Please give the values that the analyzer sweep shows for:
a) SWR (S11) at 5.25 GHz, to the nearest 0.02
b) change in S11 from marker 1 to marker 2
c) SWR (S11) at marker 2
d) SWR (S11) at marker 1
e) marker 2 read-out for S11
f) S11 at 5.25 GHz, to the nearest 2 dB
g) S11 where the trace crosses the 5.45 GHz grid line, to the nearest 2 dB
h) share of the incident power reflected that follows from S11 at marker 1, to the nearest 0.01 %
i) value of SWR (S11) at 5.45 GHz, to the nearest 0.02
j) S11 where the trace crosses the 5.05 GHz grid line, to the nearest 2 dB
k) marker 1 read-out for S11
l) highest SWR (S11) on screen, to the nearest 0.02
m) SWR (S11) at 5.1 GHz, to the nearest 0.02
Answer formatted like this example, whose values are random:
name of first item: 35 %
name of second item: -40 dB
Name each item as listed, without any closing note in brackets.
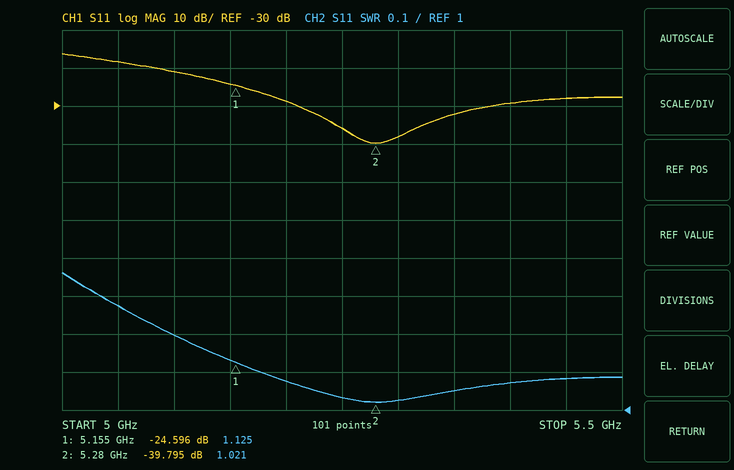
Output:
SWR (S11) at 5.25 GHz, to the nearest 0.02: 1.04
change in S11 from marker 1 to marker 2: -15.199 dB
SWR (S11) at marker 2: 1.021
SWR (S11) at marker 1: 1.125
marker 2 read-out for S11: -39.795 dB
S11 at 5.25 GHz, to the nearest 2 dB: -36 dB
S11 where the trace crosses the 5.45 GHz grid line, to the nearest 2 dB: -28 dB
share of the incident power reflected that follows from S11 at marker 1, to the nearest 0.01 %: 0.35 %
value of SWR (S11) at 5.45 GHz, to the nearest 0.02: 1.08
S11 where the trace crosses the 5.05 GHz grid line, to the nearest 2 dB: -18 dB
marker 1 read-out for S11: -24.596 dB
highest SWR (S11) on screen, to the nearest 0.02: 1.36
SWR (S11) at 5.1 GHz, to the nearest 0.02: 1.20
